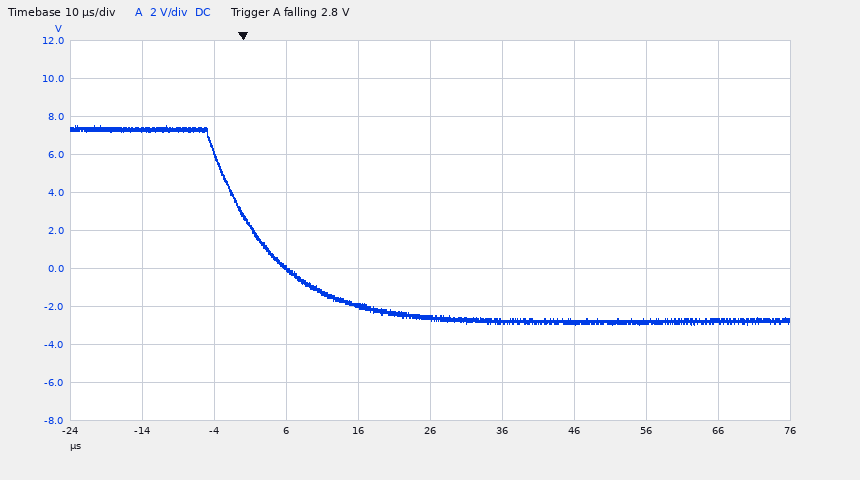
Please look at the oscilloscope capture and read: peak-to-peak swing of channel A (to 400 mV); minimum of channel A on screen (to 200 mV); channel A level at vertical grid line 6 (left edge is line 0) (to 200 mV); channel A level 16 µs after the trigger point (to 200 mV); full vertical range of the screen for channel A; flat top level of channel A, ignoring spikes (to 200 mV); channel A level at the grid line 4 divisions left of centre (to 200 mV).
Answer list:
10.4 V
-3.0 V
-2.8 V
-2.0 V
20 V
7.4 V
7.4 V
